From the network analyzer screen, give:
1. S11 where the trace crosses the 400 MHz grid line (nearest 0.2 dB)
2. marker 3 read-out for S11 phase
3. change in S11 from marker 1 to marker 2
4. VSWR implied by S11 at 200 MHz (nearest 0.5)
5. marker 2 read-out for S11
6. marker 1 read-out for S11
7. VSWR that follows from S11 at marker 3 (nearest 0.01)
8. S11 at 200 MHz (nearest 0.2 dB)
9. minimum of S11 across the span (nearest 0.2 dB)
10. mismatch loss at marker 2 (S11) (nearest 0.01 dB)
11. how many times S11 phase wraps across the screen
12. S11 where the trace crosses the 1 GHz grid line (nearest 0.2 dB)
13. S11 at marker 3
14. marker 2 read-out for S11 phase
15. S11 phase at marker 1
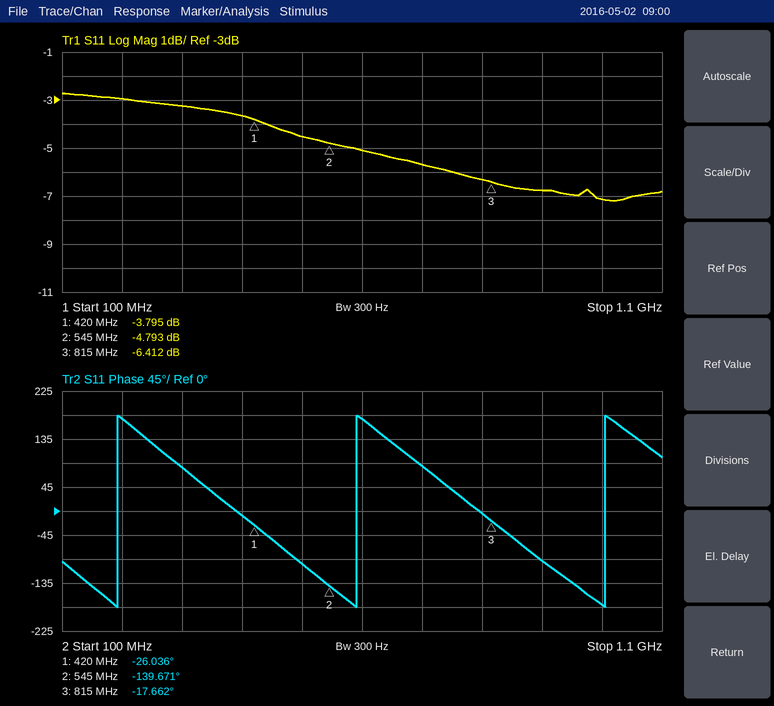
-3.6 dB
-17.662°
-0.998 dB
6.0
-4.793 dB
-3.795 dB
2.83
-3.0 dB
-7.2 dB
1.75 dB
3
-7.2 dB
-6.412 dB
-139.671°
-26.036°
